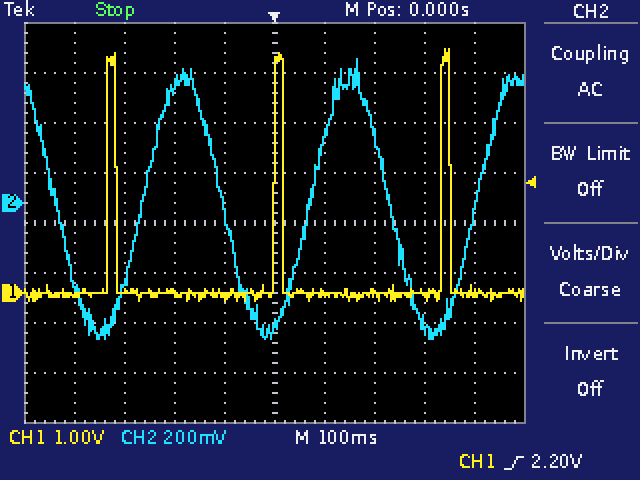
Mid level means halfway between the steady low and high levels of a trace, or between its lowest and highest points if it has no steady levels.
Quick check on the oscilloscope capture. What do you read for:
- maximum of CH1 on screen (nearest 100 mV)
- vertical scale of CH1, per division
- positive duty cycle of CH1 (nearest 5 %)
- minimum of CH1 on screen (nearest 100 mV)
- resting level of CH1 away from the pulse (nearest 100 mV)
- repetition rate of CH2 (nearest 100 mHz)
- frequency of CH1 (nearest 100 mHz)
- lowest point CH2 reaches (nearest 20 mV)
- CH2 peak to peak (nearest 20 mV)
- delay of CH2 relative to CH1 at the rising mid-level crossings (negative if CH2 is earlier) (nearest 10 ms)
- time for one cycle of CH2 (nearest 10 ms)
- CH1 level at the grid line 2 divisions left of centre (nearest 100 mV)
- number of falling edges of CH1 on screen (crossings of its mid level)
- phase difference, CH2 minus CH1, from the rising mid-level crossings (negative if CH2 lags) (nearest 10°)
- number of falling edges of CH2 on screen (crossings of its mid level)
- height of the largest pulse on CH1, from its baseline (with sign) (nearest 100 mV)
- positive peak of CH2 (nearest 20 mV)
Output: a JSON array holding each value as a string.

["4.9 V", "1 V", "5 %", "-200 mV", "0.0 V", "3.0 Hz", "3.0 Hz", "-540 mV", "1.12 V", "+70 ms", "330 ms", "0.0 V", "3", "-80°", "3", "+4.9 V", "580 mV"]
